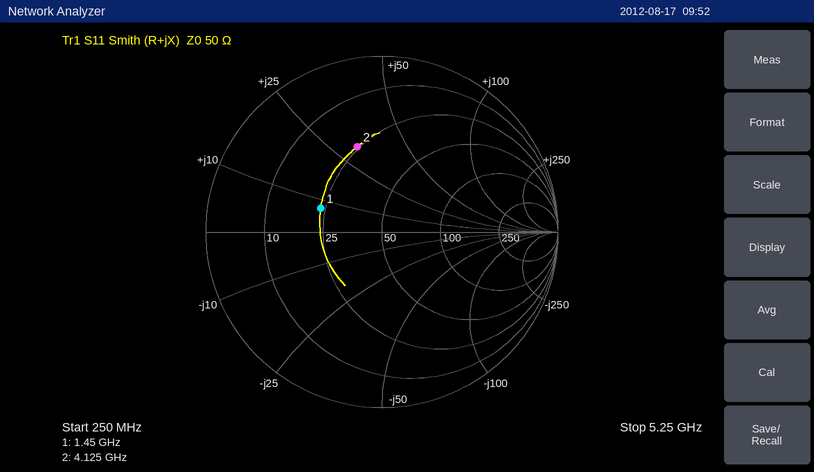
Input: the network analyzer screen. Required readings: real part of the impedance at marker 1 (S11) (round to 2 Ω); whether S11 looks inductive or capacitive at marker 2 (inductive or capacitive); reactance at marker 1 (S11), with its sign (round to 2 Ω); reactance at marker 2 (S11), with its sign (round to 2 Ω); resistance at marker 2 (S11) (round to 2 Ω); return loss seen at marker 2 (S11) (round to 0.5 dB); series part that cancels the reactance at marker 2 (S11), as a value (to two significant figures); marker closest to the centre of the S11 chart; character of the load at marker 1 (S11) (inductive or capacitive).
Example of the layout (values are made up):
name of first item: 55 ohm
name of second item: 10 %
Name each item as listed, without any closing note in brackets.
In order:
real part of the impedance at marker 1 (S11): 24 Ω
whether S11 looks inductive or capacitive at marker 2: inductive
reactance at marker 1 (S11), with its sign: +8 Ω
reactance at marker 2 (S11), with its sign: +32 Ω
resistance at marker 2 (S11): 24 Ω
return loss seen at marker 2 (S11): 6.0 dB
series part that cancels the reactance at marker 2 (S11), as a value: 1.2 pF
marker closest to the centre of the S11 chart: marker 1
character of the load at marker 1 (S11): inductive
